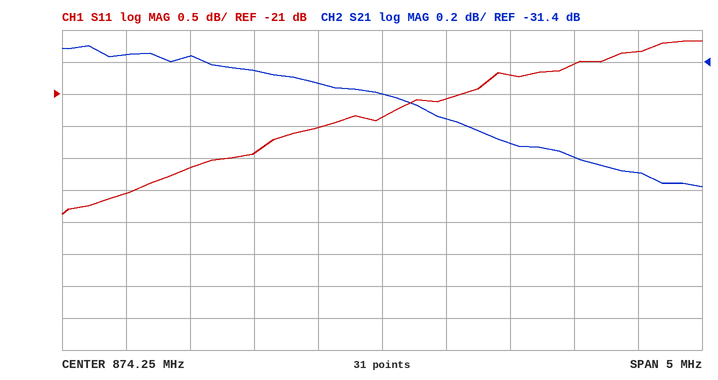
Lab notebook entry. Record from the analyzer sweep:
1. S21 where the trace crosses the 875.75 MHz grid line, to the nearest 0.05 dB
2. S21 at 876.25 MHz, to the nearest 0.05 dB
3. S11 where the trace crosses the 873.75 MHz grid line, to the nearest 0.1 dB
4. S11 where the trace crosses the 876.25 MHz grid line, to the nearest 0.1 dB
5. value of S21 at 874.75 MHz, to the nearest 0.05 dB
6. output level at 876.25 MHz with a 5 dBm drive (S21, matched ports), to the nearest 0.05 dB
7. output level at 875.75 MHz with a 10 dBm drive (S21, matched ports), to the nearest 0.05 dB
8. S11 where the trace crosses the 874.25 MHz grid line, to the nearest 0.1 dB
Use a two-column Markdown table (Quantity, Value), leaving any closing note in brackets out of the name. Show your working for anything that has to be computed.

| Quantity | Value |
|---|---|
| S21 where the trace crosses the 875.75 MHz grid line, to the nearest 0.05 dB | -32.00 dB |
| S21 at 876.25 MHz, to the nearest 0.05 dB | -32.10 dB |
| S11 where the trace crosses the 873.75 MHz grid line, to the nearest 0.1 dB | -21.5 dB |
| S11 where the trace crosses the 876.25 MHz grid line, to the nearest 0.1 dB | -20.3 dB |
| value of S21 at 874.75 MHz, to the nearest 0.05 dB | -31.75 dB |
| output level at 876.25 MHz with a 5 dBm drive (S21, matched ports), to the nearest 0.05 dB | 5 dBm + (-32.10 dB) = -27.10 dBm |
| output level at 875.75 MHz with a 10 dBm drive (S21, matched ports), to the nearest 0.05 dB | 10 dBm + (-32.00 dB) = -22.00 dBm |
| S11 where the trace crosses the 874.25 MHz grid line, to the nearest 0.1 dB | -21.4 dB |
